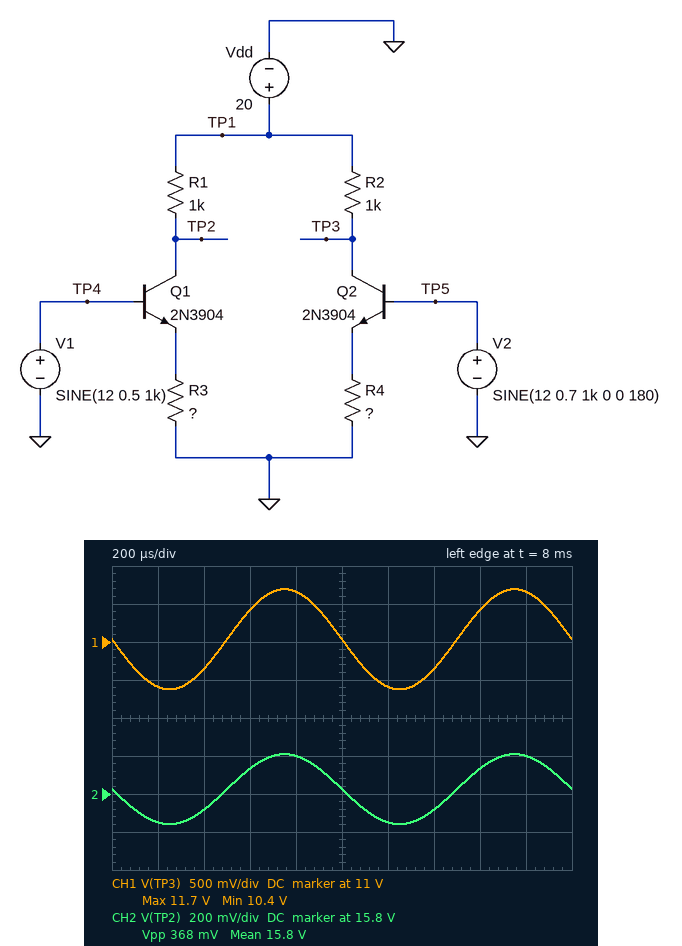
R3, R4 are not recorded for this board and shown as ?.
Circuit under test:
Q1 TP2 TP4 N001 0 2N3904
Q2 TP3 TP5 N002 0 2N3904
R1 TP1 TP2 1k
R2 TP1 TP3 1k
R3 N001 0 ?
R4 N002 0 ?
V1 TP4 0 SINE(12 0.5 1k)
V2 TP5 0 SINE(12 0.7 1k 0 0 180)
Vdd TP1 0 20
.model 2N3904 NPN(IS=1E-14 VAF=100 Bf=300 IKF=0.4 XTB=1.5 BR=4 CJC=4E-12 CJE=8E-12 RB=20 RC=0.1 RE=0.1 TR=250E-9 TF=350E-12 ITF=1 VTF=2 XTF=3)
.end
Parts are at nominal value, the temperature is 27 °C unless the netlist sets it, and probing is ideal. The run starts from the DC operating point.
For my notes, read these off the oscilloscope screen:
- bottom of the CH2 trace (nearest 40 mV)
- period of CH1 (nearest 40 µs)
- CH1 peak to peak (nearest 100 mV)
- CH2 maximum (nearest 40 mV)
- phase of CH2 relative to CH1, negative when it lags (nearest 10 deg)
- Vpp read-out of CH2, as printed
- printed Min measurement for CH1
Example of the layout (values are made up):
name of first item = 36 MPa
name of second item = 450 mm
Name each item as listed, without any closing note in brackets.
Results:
bottom of the CH2 trace = 15.64 V
period of CH1 = 1.00 ms
CH1 peak to peak = 1.3 V
CH2 maximum = 16.00 V
phase of CH2 relative to CH1, negative when it lags = 0 deg
Vpp read-out of CH2, as printed = 368 mV
printed Min measurement for CH1 = 10.4 V
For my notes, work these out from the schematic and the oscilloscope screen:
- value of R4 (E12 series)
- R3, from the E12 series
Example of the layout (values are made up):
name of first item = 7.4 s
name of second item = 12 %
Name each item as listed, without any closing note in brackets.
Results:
value of R4 = 560 Ω
R3, from the E12 series = 2.7 kΩ
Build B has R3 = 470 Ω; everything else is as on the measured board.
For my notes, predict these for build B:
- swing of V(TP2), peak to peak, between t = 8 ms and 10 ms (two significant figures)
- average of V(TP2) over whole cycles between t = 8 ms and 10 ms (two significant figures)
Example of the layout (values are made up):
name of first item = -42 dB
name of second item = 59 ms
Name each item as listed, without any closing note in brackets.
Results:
swing of V(TP2), peak to peak, between t = 8 ms and 10 ms = 940 mV
average of V(TP2) over whole cycles between t = 8 ms and 10 ms = 11 V
